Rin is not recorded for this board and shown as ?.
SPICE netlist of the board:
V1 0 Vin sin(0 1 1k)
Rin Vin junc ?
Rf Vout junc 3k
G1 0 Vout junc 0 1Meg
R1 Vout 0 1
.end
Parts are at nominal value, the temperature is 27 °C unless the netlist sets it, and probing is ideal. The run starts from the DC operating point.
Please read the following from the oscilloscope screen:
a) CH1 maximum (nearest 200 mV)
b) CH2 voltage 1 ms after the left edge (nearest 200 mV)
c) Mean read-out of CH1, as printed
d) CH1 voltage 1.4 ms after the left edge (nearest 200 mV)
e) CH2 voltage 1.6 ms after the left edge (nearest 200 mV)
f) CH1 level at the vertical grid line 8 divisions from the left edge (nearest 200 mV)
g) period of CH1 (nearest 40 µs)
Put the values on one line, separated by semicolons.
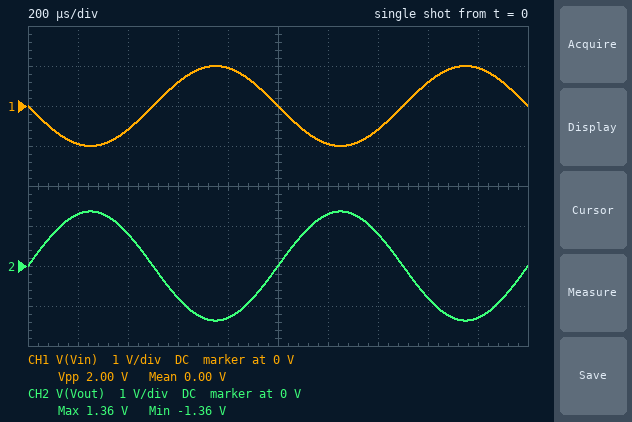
1.0 V; 0 V; 0.00 V; -600 mV; -800 mV; 600 mV; 1.00 ms
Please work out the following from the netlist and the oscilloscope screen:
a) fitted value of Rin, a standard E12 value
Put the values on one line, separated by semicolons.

2.2 kΩ
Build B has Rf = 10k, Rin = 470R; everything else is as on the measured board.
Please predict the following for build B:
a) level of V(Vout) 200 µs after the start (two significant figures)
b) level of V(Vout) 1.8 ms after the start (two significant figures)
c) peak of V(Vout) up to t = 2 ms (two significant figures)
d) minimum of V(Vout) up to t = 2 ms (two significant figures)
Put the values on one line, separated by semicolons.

20 V; -20 V; 21 V; -21 V
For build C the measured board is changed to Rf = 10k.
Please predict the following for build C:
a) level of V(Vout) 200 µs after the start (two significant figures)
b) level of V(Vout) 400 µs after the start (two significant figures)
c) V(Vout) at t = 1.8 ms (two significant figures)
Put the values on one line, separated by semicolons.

4.3 V; 2.7 V; -4.3 V
